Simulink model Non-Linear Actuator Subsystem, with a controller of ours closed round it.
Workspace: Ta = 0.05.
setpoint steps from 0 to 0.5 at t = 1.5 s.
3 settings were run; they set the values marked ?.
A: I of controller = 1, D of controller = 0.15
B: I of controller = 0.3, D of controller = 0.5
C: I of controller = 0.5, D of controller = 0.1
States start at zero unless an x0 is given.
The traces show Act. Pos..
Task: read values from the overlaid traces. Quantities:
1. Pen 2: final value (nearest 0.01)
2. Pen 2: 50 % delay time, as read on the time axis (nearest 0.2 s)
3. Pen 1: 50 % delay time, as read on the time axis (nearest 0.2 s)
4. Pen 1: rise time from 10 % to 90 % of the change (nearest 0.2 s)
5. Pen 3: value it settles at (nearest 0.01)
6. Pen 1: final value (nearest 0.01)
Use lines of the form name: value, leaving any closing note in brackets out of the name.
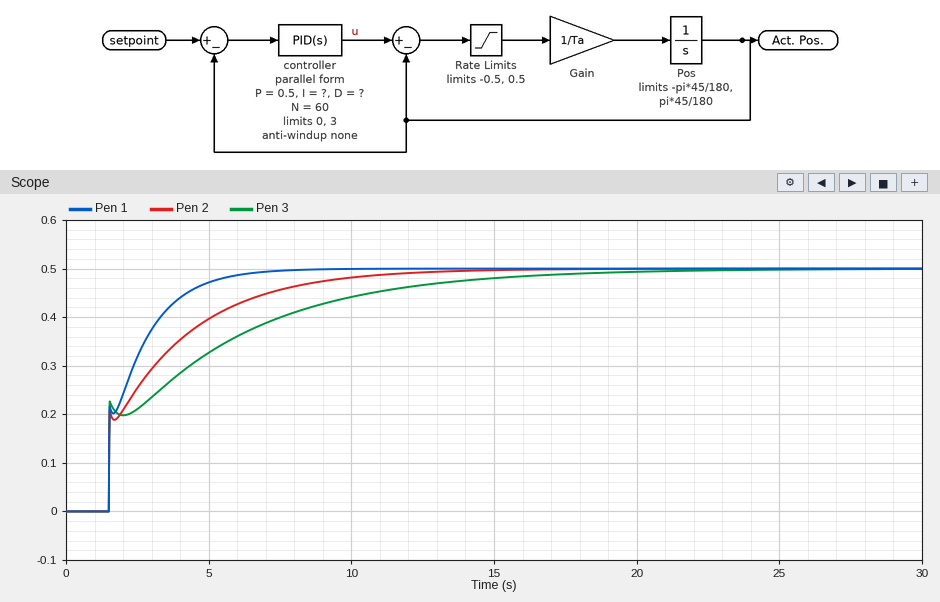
Pen 2: final value: 0.50
Pen 2: 50 % delay time, as read on the time axis: 2.4 s
Pen 1: 50 % delay time, as read on the time axis: 2.0 s
Pen 1: rise time from 10 % to 90 % of the change: 2.8 s
Pen 3: value it settles at: 0.50
Pen 1: final value: 0.50
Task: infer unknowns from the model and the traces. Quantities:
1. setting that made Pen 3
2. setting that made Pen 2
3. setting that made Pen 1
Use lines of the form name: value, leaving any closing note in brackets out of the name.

setting that made Pen 3: B
setting that made Pen 2: C
setting that made Pen 1: A
